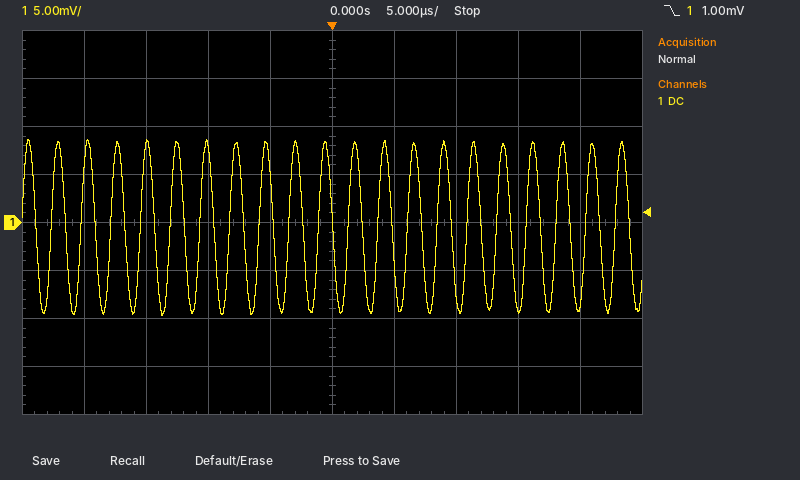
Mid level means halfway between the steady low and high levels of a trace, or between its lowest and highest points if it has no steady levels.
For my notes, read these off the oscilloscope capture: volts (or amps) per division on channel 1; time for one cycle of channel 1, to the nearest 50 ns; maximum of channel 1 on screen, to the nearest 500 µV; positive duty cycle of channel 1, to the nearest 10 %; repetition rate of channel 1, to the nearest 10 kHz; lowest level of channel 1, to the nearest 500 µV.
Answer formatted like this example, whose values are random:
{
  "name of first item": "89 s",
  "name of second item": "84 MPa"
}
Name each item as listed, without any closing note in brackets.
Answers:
{
  "volts (or amps) per division on channel 1": "5 mV",
  "time for one cycle of channel 1, to the nearest 50 ns": "2.40 µs",
  "maximum of channel 1 on screen, to the nearest 500 µV": "8.5 mV",
  "positive duty cycle of channel 1, to the nearest 10 %": "50 %",
  "repetition rate of channel 1, to the nearest 10 kHz": "420 kHz",
  "lowest level of channel 1, to the nearest 500 µV": "-9.5 mV"
}
